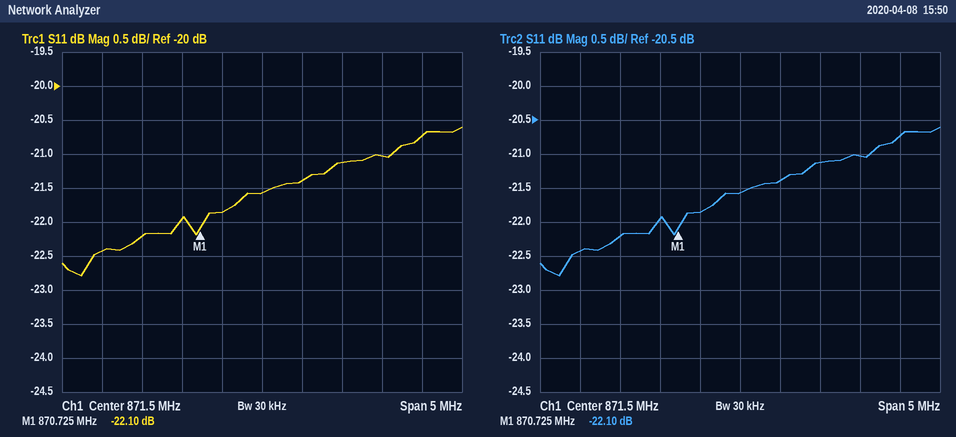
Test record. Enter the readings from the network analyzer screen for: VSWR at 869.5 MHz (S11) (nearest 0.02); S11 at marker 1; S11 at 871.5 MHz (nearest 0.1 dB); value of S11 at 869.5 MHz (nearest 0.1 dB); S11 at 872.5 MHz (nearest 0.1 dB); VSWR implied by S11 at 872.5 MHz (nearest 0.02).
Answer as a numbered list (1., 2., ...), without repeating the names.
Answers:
1. 1.16
2. -22.10 dB
3. -21.6 dB
4. -22.4 dB
5. -21.1 dB
6. 1.20
